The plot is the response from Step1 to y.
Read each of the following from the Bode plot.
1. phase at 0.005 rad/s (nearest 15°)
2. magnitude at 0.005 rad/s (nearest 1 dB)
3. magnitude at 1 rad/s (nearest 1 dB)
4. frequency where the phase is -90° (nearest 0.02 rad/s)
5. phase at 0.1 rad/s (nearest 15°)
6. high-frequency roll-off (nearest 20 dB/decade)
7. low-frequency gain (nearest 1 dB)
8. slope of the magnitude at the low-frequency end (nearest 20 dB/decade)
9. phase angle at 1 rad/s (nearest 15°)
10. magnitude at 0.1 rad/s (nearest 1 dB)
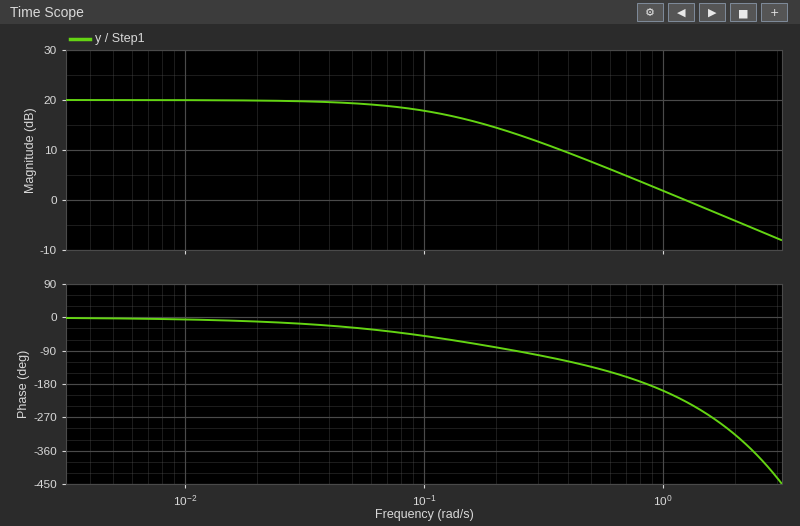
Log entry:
0°
20 dB
2 dB
0.24 rad/s
-45°
-20 dB/decade
20 dB
0 dB/decade
-195°
18 dB
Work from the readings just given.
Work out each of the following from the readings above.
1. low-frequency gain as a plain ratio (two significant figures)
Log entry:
10
